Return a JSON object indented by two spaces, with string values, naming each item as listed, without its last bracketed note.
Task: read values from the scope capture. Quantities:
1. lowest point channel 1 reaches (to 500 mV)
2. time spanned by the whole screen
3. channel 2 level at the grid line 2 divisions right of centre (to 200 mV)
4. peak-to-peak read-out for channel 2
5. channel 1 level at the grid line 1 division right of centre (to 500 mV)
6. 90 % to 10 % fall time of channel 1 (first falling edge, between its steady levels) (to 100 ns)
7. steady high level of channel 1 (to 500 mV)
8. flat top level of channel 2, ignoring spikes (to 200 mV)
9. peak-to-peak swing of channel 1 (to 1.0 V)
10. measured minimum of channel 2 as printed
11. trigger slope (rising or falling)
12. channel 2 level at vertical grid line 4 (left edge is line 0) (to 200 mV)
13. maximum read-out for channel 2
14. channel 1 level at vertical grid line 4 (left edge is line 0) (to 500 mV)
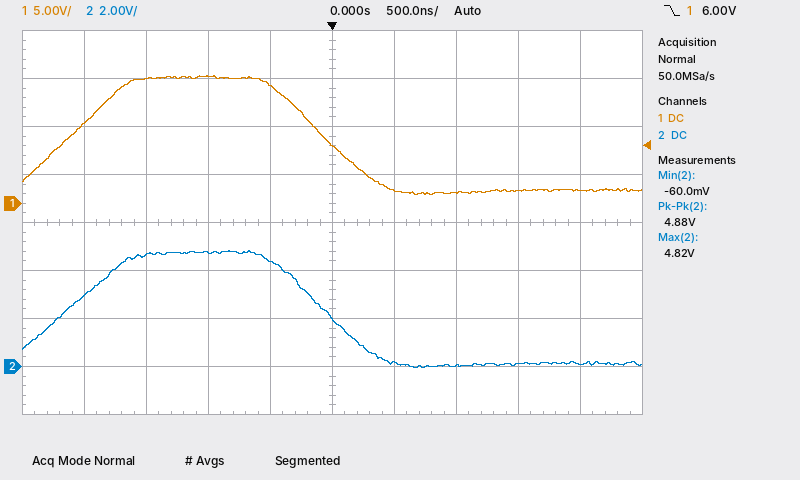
{
  "lowest point channel 1 reaches": "1.0 V",
  "time spanned by the whole screen": "5 µs",
  "channel 2 level at the grid line 2 divisions right of centre": "0.0 V",
  "peak-to-peak read-out for channel 2": "4.88 V",
  "channel 1 level at the grid line 1 division right of centre": "1.5 V",
  "90 % to 10 % fall time of channel 1 (first falling edge, between its steady levels)": "800 ns",
  "steady high level of channel 1": "13.0 V",
  "flat top level of channel 2, ignoring spikes": "4.8 V",
  "peak-to-peak swing of channel 1": "12.0 V",
  "measured minimum of channel 2 as printed": "-60.0 mV",
  "trigger slope": "falling",
  "channel 2 level at vertical grid line 4 (left edge is line 0)": "4.4 V",
  "maximum read-out for channel 2": "4.82 V",
  "channel 1 level at vertical grid line 4 (left edge is line 0)": "12.5 V"
}
